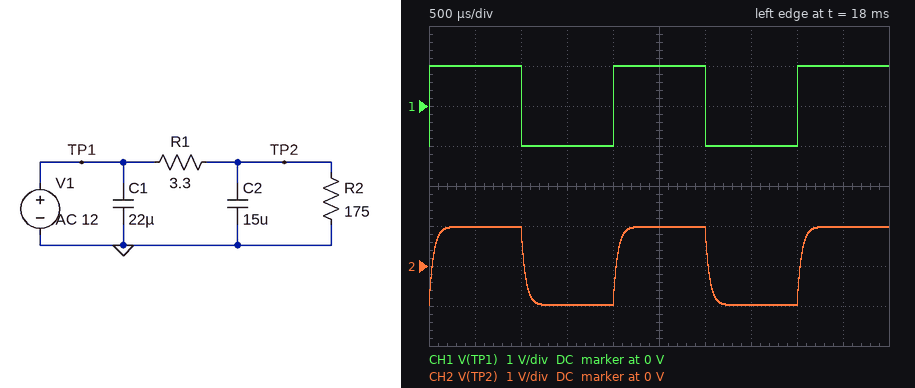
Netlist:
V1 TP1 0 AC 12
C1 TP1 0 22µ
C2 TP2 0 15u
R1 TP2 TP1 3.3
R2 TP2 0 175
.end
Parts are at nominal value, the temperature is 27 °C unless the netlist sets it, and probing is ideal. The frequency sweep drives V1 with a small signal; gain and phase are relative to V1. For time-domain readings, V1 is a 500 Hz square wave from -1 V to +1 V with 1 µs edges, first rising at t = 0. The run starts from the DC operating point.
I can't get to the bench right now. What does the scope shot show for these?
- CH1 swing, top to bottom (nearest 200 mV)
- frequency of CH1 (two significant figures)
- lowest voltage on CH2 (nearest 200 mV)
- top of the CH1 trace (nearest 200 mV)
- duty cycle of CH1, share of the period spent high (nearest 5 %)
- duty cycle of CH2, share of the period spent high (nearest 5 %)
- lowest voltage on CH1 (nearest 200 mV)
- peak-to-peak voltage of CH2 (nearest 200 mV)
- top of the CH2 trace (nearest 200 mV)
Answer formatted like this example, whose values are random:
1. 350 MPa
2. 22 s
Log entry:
1. 2.0 V
2. 500 Hz
3. -1.0 V
4. 1.0 V
5. 50 %
6. 50 %
7. -1.0 V
8. 2.0 V
9. 1.0 V
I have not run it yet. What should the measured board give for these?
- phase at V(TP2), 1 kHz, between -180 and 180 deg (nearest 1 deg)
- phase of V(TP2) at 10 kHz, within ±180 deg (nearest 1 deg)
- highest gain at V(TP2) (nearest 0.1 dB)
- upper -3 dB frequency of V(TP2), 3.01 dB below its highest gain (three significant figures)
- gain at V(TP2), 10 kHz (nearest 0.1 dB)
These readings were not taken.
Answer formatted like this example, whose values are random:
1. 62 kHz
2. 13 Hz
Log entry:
1. -17 deg
2. -72 deg
3. -0.2 dB
4. 3.28 kHz
5. -10.3 dB
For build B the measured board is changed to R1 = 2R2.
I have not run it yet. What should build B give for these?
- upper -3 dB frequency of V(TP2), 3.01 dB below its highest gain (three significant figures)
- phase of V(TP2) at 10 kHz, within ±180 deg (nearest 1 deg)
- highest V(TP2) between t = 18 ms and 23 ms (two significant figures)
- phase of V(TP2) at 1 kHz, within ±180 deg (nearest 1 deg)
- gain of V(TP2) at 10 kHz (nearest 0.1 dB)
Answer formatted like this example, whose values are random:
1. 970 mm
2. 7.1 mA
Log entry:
1. 4.88 kHz
2. -64 deg
3. 990 mV
4. -12 deg
5. -7.3 dB
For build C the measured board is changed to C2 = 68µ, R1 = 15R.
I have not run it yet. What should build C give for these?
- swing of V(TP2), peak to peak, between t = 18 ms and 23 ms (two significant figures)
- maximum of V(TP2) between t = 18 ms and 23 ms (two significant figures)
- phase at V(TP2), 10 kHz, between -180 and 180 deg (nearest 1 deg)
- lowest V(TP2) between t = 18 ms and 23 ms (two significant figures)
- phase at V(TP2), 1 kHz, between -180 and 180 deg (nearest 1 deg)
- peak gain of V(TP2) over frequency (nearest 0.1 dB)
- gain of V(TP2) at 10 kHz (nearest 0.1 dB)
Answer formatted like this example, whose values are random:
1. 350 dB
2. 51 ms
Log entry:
1. 900 mV
2. 450 mV
3. -89 deg
4. -450 mV
5. -80 deg
6. -0.7 dB
7. -36.1 dB
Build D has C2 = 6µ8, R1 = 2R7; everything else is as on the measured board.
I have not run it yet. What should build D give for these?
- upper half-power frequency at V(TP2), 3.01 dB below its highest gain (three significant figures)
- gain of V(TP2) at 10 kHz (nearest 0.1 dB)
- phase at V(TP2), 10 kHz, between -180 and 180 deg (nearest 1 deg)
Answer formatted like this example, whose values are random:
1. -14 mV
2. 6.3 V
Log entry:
1. 8.80 kHz
2. -3.7 dB
3. -49 deg
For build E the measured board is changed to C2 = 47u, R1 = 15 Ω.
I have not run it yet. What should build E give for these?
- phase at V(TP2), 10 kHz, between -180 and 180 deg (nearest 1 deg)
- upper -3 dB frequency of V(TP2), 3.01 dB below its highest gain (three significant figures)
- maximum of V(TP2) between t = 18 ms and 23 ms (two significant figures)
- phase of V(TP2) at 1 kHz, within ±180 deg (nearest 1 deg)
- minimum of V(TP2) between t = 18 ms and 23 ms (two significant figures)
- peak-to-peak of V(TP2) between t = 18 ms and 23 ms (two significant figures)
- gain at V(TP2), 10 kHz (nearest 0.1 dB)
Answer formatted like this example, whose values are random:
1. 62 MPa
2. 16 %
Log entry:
1. -89 deg
2. 245 Hz
3. 600 mV
4. -76 deg
5. -600 mV
6. 1.2 V
7. -32.9 dB
